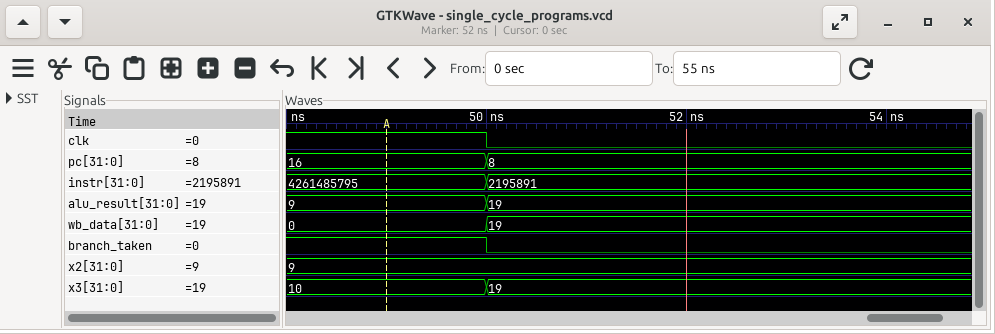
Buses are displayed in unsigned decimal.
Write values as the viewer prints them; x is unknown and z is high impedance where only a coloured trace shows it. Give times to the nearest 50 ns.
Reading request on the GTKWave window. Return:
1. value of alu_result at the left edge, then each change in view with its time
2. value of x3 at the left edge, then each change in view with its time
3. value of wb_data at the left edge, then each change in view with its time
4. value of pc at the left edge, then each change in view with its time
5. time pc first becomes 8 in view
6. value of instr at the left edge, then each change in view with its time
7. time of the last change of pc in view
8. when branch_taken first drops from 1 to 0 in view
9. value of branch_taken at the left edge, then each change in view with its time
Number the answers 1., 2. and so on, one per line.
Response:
1. 9, 19 at 50 ns
2. 10, 19 at 50 ns
3. 0, 19 at 50 ns
4. 16, 8 at 50 ns
5. 50 ns
6. 4261485795, 2195891 at 50 ns
7. 50 ns
8. 50 ns
9. 1, 0 at 50 ns
